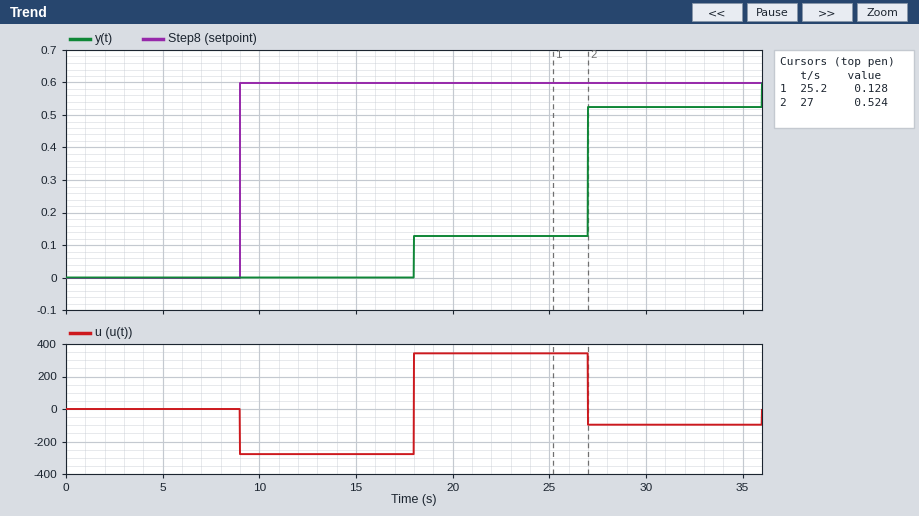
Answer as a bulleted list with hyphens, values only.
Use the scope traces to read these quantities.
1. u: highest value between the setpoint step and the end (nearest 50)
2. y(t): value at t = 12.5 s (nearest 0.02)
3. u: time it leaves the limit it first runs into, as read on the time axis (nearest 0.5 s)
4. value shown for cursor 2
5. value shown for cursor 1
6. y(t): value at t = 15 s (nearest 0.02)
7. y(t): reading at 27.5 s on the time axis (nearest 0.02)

- 350
- 0.00
- 18.0 s
- 0.524
- 0.128
- 0.00
- 0.52
